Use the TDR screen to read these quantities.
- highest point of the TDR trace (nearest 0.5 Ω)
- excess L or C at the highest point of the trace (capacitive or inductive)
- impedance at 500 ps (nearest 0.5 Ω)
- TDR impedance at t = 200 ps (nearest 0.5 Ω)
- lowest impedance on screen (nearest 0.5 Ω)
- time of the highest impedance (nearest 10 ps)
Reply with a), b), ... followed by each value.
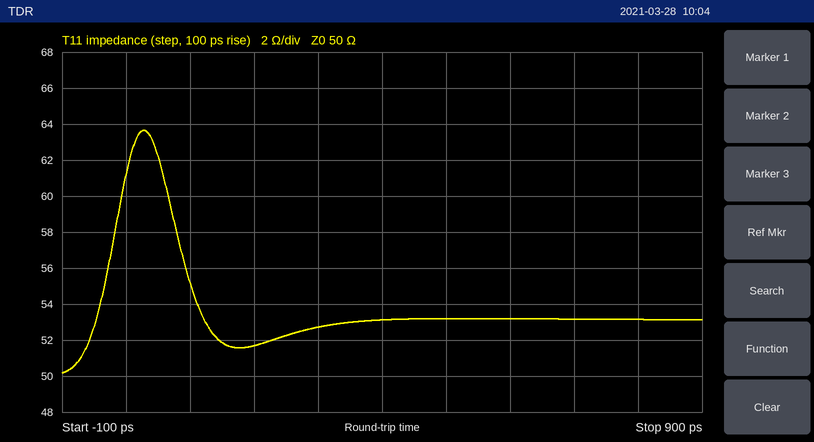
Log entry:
a) 63.5 Ω
b) inductive
c) 53.0 Ω
d) 51.5 Ω
e) 50.0 Ω
f) 30 ps
